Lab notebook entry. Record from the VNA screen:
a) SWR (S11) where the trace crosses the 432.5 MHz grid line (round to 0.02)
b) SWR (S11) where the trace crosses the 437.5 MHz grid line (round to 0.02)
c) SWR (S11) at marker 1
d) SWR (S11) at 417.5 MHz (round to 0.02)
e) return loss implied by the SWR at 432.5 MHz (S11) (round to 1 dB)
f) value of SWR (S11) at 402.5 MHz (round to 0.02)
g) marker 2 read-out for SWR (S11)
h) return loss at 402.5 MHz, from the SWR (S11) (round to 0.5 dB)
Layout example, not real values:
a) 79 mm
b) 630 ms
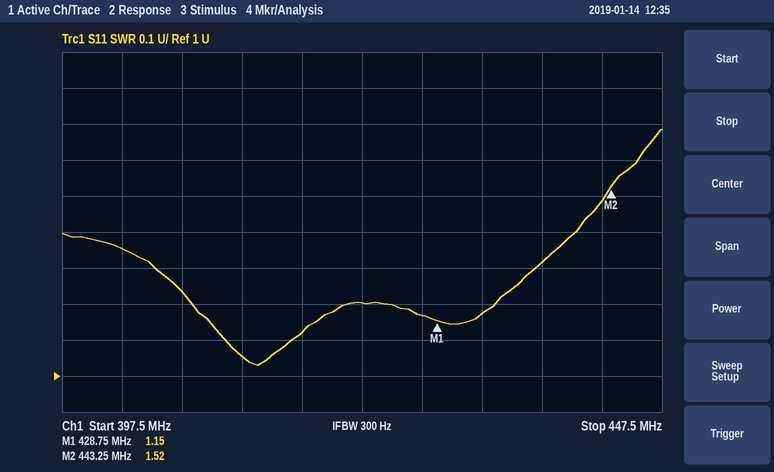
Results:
a) 1.18
b) 1.32
c) 1.15
d) 1.12
e) 22 dB
f) 1.36
g) 1.52
h) 16.5 dB
